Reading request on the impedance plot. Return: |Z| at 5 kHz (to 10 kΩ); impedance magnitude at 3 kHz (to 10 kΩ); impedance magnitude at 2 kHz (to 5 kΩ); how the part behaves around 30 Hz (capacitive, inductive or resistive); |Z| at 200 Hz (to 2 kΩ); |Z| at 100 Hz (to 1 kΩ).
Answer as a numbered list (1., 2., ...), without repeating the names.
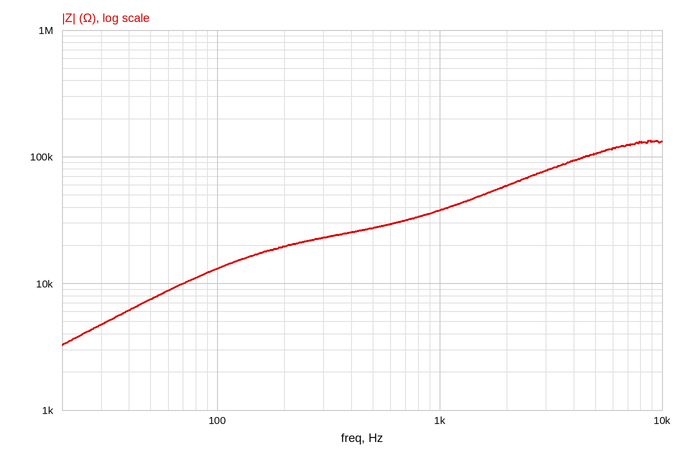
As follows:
1. 110 kΩ
2. 80 kΩ
3. 60 kΩ
4. inductive
5. 20 kΩ
6. 13 kΩ
